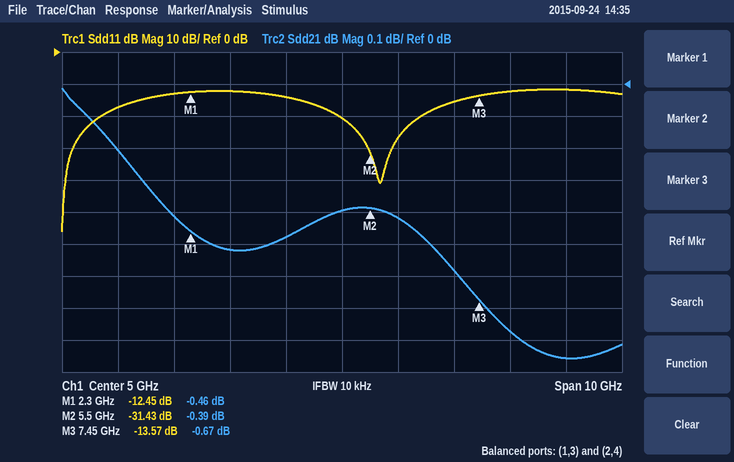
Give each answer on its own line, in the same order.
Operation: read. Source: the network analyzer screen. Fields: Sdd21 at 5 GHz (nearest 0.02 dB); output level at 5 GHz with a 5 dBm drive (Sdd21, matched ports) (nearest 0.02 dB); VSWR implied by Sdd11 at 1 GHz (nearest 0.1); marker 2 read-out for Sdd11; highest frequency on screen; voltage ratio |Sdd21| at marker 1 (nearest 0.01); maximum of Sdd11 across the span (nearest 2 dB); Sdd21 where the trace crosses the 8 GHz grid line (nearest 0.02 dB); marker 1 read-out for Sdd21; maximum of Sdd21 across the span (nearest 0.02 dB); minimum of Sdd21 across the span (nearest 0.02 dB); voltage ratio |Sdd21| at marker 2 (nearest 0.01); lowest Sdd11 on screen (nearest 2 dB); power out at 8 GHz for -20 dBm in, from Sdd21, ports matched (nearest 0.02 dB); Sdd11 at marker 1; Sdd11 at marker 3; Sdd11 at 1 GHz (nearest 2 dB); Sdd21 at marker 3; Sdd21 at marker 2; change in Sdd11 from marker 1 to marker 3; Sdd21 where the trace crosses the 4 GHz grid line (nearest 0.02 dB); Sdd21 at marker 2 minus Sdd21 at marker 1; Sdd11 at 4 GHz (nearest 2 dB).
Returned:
-0.40 dB
4.60 dBm
1.3
-31.43 dB
10 GHz
0.95
-12 dB
-0.78 dB
-0.46 dB
-0.02 dB
-0.86 dB
0.96
-56 dB
-20.78 dBm
-12.45 dB
-13.57 dB
-18 dB
-0.67 dB
-0.39 dB
-1.12 dB
-0.48 dB
0.07 dB
-14 dB
